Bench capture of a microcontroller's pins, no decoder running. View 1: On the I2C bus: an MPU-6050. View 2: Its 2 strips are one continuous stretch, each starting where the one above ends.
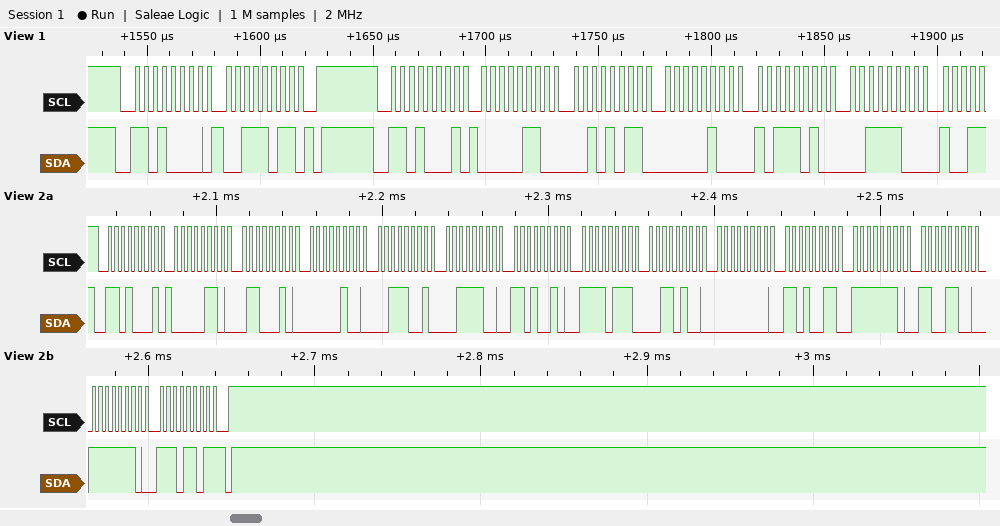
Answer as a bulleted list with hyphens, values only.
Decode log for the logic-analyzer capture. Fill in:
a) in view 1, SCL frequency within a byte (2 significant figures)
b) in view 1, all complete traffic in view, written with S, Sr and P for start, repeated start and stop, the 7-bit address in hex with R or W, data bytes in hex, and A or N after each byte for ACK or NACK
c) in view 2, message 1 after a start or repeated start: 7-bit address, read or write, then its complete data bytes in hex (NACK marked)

- 250 kHz
- S 68W A 3B A P S 68R A 06 A 2B A 04 A BA A 3C A
- 0x68 read: 06 62 04 39 3C D2 F7 34 00 D3 FE CC FE ED NACK
